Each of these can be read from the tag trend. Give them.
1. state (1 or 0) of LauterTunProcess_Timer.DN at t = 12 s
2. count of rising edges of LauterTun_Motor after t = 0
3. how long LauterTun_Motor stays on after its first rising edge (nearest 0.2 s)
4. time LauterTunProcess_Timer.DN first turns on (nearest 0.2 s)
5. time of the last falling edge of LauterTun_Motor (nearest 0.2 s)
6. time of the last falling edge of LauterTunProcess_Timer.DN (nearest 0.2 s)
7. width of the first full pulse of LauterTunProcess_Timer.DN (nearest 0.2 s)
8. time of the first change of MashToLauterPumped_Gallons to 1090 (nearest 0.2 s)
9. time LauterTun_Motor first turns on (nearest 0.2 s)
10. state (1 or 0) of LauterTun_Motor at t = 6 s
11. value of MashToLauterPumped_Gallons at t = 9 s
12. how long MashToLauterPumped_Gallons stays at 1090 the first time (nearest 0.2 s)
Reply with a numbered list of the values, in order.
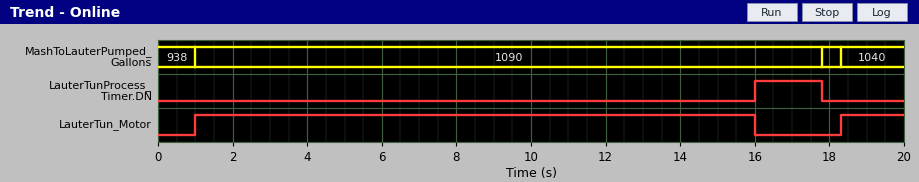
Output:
1. 0
2. 2
3. 15.0 s
4. 16.0 s
5. 16.0 s
6. 17.8 s
7. 1.8 s
8. 1.0 s
9. 1.0 s
10. 1
11. 1090
12. 16.8 s
